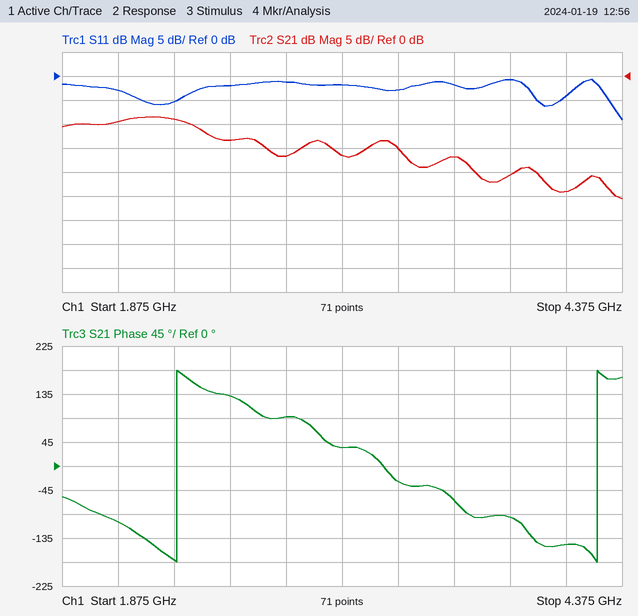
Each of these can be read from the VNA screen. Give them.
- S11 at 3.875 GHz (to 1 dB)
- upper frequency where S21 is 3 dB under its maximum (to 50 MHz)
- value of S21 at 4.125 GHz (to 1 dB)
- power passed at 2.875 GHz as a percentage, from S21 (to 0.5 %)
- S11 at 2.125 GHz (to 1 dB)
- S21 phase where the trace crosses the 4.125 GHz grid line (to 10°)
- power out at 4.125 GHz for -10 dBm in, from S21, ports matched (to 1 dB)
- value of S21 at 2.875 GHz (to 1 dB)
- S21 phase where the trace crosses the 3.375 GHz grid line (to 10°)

-1 dB
2.50 GHz
-24 dB
2.0 %
-3 dB
-150°
-34 dBm
-17 dB
-30°
